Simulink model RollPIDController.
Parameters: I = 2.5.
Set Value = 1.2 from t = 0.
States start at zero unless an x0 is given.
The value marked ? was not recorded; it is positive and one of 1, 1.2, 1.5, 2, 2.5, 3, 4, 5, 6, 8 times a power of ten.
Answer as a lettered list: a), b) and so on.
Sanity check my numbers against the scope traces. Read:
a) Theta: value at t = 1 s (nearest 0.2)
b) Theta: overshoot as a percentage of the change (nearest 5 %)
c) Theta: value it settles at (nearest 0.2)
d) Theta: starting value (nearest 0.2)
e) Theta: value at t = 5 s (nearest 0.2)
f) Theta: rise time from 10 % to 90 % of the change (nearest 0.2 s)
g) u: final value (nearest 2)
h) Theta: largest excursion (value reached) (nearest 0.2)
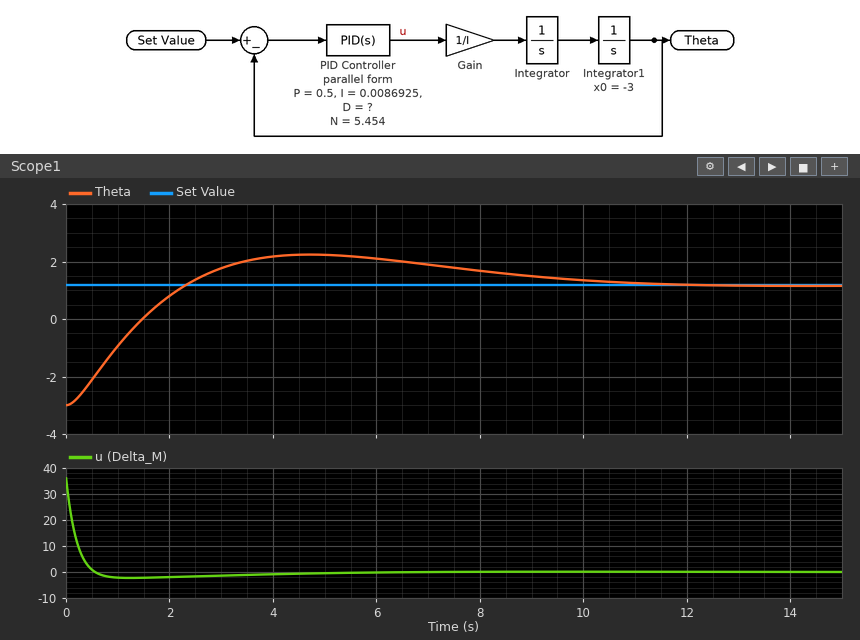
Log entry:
a) -1.0
b) 25 %
c) 1.2
d) -3.0
e) 2.2
f) 1.6 s
g) 0
h) 2.2
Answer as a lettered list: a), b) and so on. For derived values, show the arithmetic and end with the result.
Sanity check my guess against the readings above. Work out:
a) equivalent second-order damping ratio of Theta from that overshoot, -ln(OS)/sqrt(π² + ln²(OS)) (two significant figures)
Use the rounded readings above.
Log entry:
a) ln(0.25) = -1.386; 1.386 / sqrt(9.870 + 1.922) = 0.40
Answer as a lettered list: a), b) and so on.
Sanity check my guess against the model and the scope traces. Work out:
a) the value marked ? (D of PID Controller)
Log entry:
a) 1.5
